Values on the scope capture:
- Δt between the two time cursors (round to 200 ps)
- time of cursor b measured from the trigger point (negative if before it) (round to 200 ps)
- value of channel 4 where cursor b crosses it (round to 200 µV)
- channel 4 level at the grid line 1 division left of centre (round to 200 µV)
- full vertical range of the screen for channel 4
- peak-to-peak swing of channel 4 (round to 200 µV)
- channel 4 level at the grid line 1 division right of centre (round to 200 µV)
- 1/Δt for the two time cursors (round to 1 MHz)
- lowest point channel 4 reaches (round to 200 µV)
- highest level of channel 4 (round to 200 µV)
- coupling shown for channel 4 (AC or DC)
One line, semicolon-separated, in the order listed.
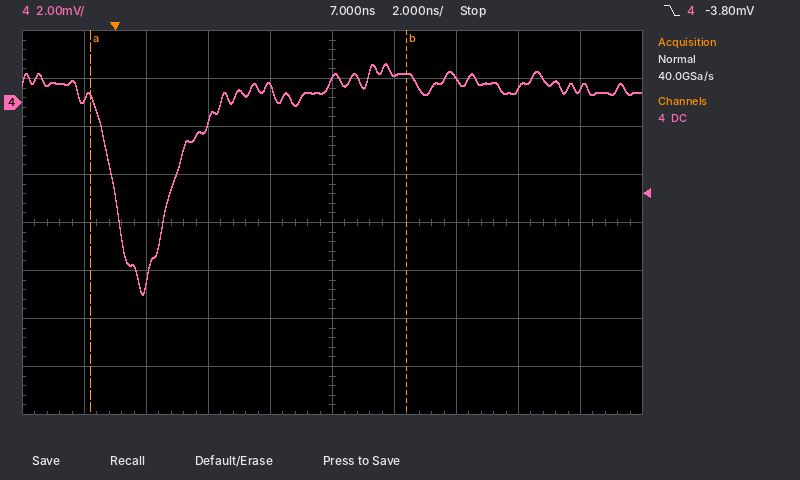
10.2 ns; +9.4 ns; 1.2 mV; 600 µV; 16 mV; 9.6 mV; 1.2 mV; 98 MHz; -8.0 mV; 1.6 mV; DC
